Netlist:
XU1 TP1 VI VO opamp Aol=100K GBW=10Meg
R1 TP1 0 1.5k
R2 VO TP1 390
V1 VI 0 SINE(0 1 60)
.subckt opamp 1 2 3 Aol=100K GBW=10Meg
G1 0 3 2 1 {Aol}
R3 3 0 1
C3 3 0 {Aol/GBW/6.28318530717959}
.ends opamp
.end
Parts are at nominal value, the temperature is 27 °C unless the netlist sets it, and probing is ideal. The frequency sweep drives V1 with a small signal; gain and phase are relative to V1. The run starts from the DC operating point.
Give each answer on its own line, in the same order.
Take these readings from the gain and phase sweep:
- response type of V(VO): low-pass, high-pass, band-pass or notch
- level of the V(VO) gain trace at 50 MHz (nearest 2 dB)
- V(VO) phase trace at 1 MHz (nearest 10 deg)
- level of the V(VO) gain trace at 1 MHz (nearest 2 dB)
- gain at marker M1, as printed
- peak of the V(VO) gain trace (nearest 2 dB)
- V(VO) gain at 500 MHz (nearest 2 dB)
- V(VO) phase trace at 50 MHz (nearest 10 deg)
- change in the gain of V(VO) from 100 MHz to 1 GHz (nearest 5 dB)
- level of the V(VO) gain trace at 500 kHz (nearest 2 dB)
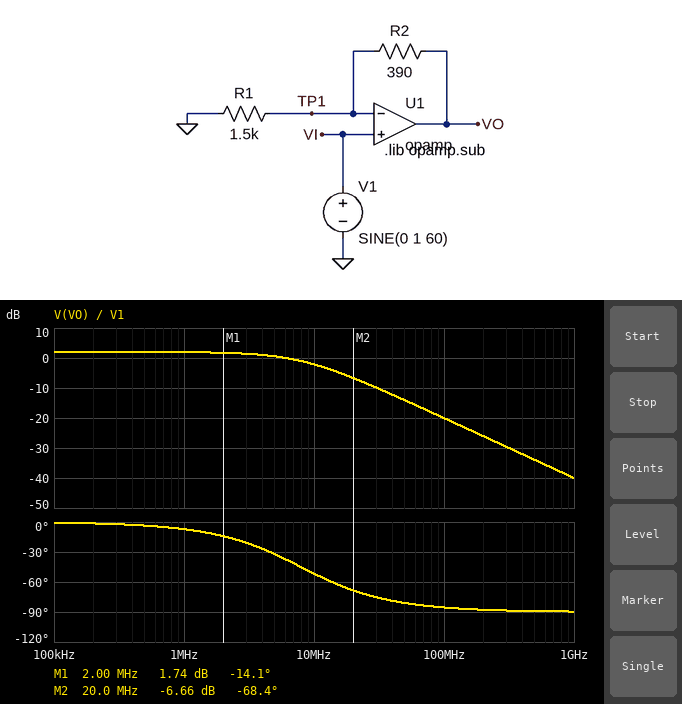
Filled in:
low-pass
-14 dB
-10 deg
2 dB
1.74 dB
2 dB
-34 dB
-80 deg
-20 dB
2 dB
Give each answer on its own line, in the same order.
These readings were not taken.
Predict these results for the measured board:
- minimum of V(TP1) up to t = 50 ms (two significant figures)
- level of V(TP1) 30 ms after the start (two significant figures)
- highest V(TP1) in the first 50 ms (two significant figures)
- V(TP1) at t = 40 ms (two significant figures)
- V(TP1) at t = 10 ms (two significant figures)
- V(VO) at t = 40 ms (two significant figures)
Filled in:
-1.0 V
-950 mV
1.0 V
590 mV
-590 mV
740 mV
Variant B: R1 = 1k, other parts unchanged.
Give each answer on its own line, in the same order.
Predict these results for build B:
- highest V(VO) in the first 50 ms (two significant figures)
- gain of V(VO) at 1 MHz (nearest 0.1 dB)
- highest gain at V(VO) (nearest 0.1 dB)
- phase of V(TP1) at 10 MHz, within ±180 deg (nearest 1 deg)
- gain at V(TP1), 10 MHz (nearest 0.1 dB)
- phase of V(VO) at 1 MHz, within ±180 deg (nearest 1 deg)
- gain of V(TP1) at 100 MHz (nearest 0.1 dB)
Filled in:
1.4 V
2.8 dB
2.9 dB
-54 deg
-4.7 dB
-8 deg
-22.9 dB
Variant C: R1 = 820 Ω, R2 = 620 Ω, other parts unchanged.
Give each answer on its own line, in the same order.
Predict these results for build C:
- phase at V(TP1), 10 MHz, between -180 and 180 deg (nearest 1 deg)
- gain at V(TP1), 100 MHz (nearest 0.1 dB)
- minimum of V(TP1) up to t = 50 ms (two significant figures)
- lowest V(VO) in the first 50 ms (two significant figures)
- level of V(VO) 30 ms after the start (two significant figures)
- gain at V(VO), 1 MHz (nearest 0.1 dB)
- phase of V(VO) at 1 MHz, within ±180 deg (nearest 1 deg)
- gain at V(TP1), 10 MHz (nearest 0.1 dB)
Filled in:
-60 deg
-24.9 dB
-1.0 V
-1.8 V
-1.7 V
4.8 dB
-10 deg
-6.1 dB
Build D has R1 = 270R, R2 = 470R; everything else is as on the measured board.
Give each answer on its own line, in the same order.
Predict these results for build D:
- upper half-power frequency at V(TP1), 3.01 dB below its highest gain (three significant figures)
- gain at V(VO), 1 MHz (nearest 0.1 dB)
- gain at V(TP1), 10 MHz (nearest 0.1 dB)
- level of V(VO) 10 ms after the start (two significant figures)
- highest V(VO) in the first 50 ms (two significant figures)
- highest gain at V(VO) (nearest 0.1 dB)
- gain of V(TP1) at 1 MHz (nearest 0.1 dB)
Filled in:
3.65 MHz
8.4 dB
-9.3 dB
-1.6 V
2.7 V
8.8 dB
-0.3 dB
